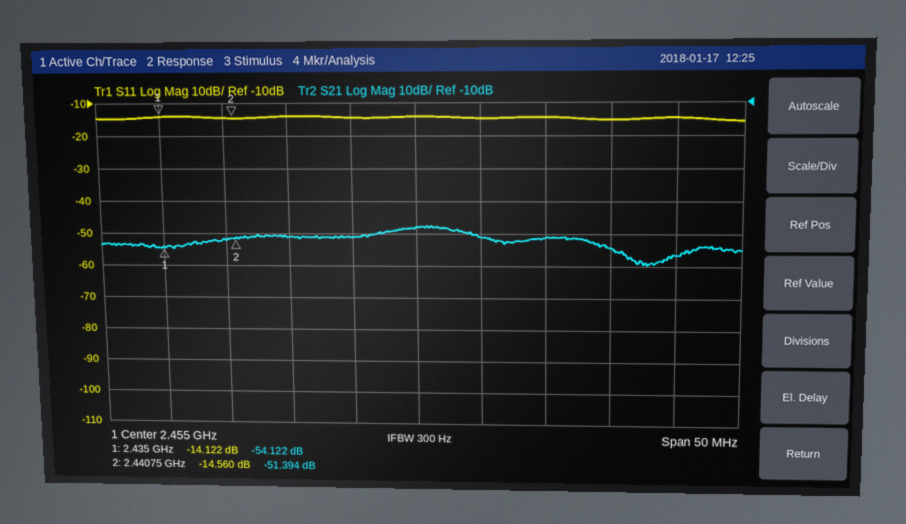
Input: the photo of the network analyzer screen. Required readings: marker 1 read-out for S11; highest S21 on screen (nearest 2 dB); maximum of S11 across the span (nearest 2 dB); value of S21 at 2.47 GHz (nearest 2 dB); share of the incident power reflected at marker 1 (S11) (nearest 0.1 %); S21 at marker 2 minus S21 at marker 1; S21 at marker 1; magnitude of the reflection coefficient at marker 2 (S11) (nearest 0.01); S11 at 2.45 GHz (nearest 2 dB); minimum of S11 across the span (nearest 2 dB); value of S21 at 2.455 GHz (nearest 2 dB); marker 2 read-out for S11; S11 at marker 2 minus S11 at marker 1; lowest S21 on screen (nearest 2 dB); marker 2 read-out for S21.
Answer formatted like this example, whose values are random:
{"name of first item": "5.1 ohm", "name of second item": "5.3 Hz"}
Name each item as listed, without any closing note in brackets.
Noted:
{"marker 1 read-out for S11": "-14.122 dB", "highest S21 on screen": "-48 dB", "maximum of S11 across the span": "-14 dB", "value of S21 at 2.47 GHz": "-54 dB", "share of the incident power reflected at marker 1 (S11)": "3.9 %", "S21 at marker 2 minus S21 at marker 1": "2.728 dB", "S21 at marker 1": "-54.122 dB", "magnitude of the reflection coefficient at marker 2 (S11)": "0.19", "S11 at 2.45 GHz": "-14 dB", "minimum of S11 across the span": "-16 dB", "value of S21 at 2.455 GHz": "-48 dB", "marker 2 read-out for S11": "-14.560 dB", "S11 at marker 2 minus S11 at marker 1": "-0.438 dB", "lowest S21 on screen": "-60 dB", "marker 2 read-out for S21": "-51.394 dB"}
